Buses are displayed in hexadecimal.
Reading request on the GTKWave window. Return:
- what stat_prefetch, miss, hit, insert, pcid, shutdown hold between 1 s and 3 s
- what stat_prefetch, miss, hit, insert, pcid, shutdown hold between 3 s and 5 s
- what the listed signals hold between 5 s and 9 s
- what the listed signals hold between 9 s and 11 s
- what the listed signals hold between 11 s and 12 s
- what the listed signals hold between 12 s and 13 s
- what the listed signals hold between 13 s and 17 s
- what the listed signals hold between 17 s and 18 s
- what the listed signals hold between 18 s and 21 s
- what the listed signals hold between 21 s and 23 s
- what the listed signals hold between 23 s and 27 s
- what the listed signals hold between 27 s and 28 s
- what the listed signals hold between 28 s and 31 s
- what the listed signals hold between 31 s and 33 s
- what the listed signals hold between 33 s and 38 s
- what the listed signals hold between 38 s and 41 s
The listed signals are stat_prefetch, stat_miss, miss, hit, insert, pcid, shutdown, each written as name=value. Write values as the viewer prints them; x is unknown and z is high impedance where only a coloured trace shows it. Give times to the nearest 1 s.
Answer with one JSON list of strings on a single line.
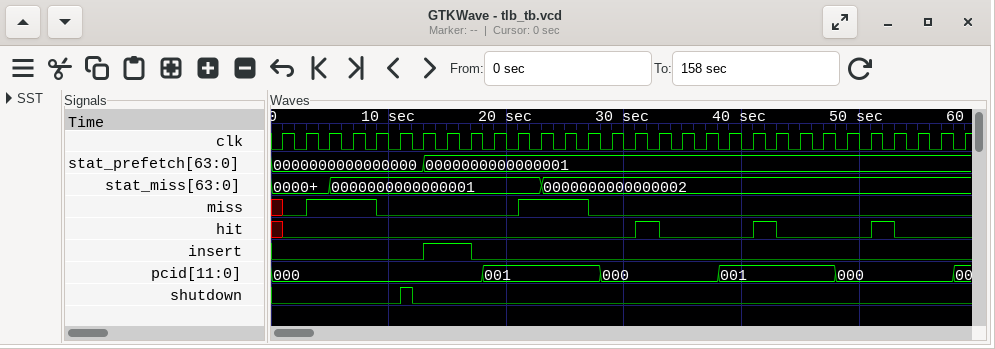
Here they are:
["stat_prefetch=0000000000000000, miss=0, hit=0, insert=0, pcid=000, shutdown=0", "stat_prefetch=0000000000000000, miss=1, hit=0, insert=0, pcid=000, shutdown=0", "stat_prefetch=0000000000000000, stat_miss=0000000000000001, miss=1, hit=0, insert=0, pcid=000, shutdown=0", "stat_prefetch=0000000000000000, stat_miss=0000000000000001, miss=0, hit=0, insert=0, pcid=000, shutdown=0", "stat_prefetch=0000000000000000, stat_miss=0000000000000001, miss=0, hit=0, insert=0, pcid=000, shutdown=1", "stat_prefetch=0000000000000000, stat_miss=0000000000000001, miss=0, hit=0, insert=0, pcid=000, shutdown=0", "stat_prefetch=0000000000000001, stat_miss=0000000000000001, miss=0, hit=0, insert=1, pcid=000, shutdown=0", "stat_prefetch=0000000000000001, stat_miss=0000000000000001, miss=0, hit=0, insert=0, pcid=000, shutdown=0", "stat_prefetch=0000000000000001, stat_miss=0000000000000001, miss=0, hit=0, insert=0, pcid=001, shutdown=0", "stat_prefetch=0000000000000001, stat_miss=0000000000000001, miss=1, hit=0, insert=0, pcid=001, shutdown=0", "stat_prefetch=0000000000000001, stat_miss=0000000000000002, miss=1, hit=0, insert=0, pcid=001, shutdown=0", "stat_prefetch=0000000000000001, stat_miss=0000000000000002, miss=0, hit=0, insert=0, pcid=001, shutdown=0", "stat_prefetch=0000000000000001, stat_miss=0000000000000002, miss=0, hit=0, insert=0, pcid=000, shutdown=0", "stat_prefetch=0000000000000001, stat_miss=0000000000000002, miss=0, hit=1, insert=0, pcid=000, shutdown=0", "stat_prefetch=0000000000000001, stat_miss=0000000000000002, miss=0, hit=0, insert=0, pcid=000, shutdown=0", "stat_prefetch=0000000000000001, stat_miss=0000000000000002, miss=0, hit=0, insert=0, pcid=001, shutdown=0"]
